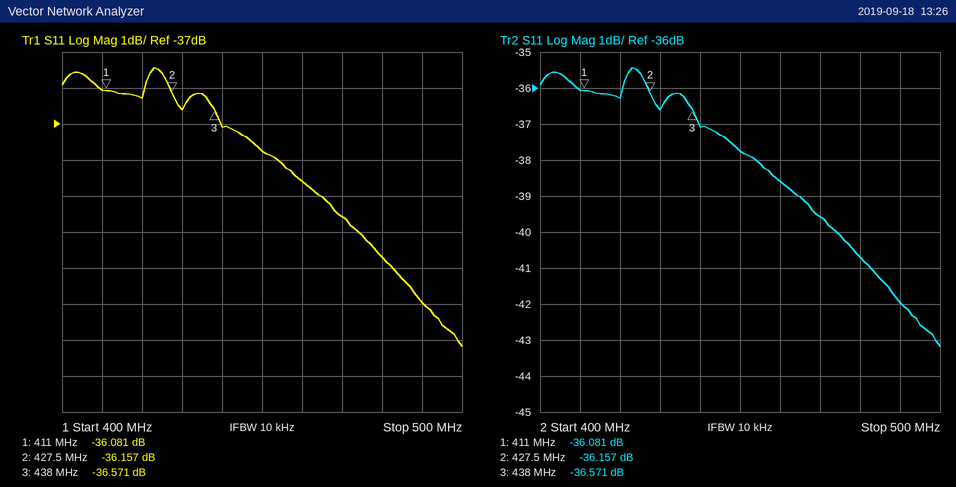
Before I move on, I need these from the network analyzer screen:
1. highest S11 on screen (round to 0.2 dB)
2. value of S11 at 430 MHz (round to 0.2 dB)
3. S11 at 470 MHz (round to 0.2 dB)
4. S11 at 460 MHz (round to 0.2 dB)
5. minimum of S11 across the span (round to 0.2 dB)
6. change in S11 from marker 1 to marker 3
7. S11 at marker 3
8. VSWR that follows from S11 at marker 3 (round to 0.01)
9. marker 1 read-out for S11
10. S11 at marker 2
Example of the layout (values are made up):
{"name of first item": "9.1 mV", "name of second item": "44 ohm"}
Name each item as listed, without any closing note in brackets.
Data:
{"highest S11 on screen": "-35.4 dB", "value of S11 at 430 MHz": "-36.6 dB", "S11 at 470 MHz": "-39.6 dB", "S11 at 460 MHz": "-38.6 dB", "minimum of S11 across the span": "-43.2 dB", "change in S11 from marker 1 to marker 3": "-0.490 dB", "S11 at marker 3": "-36.571 dB", "VSWR that follows from S11 at marker 3": "1.03", "marker 1 read-out for S11": "-36.081 dB", "S11 at marker 2": "-36.157 dB"}
